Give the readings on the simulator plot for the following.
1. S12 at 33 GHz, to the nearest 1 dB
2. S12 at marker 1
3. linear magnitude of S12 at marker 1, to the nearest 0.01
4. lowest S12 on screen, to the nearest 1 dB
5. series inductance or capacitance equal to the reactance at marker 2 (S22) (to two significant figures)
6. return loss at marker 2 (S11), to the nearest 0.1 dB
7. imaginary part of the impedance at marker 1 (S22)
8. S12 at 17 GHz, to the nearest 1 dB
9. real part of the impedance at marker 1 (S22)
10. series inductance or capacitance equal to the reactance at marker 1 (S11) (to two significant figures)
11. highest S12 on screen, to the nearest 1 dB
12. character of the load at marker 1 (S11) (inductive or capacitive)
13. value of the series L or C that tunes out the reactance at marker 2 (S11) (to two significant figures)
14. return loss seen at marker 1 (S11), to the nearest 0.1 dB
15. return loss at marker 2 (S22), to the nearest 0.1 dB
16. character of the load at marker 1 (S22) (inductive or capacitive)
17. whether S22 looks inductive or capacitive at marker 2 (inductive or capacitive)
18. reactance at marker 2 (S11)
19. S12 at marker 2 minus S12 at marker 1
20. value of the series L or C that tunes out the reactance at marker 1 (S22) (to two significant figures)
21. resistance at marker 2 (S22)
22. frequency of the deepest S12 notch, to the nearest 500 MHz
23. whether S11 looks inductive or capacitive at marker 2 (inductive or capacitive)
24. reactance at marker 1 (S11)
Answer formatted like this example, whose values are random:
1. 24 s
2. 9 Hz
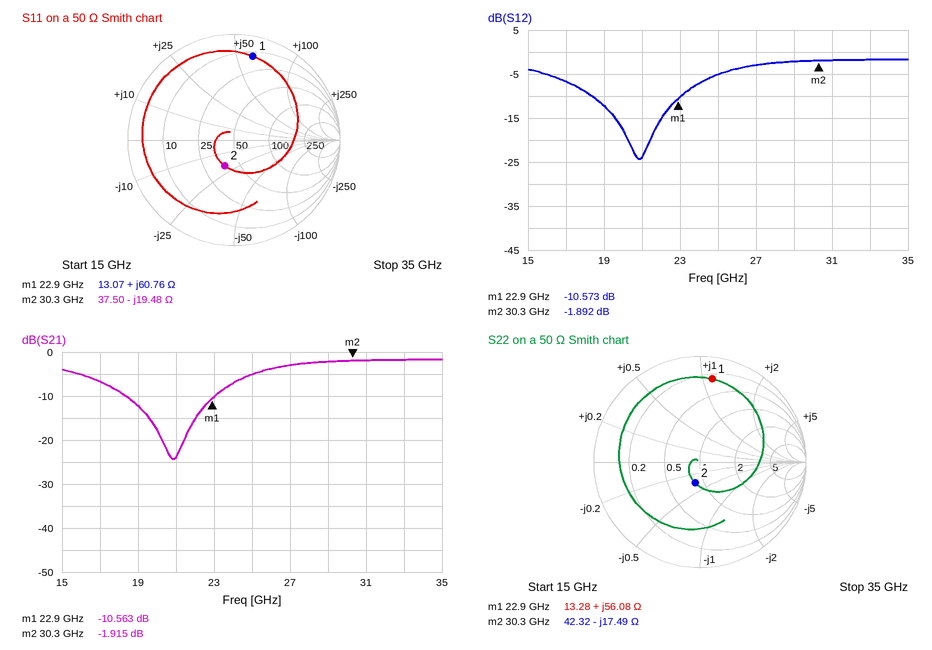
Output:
1. -2 dB
2. -10.573 dB
3. 0.30
4. -24 dB
5. 300 fF
6. 11.8 dB
7. +56.08 Ω
8. -7 dB
9. 13.28 Ω
10. 420 pH
11. -2 dB
12. inductive
13. 100 pH
14. 1.8 dB
15. 13.8 dB
16. inductive
17. capacitive
18. -19.48 Ω
19. 8.681 dB
20. 120 fF
21. 42.32 Ω
22. 21.0 GHz
23. capacitive
24. +60.76 Ω
